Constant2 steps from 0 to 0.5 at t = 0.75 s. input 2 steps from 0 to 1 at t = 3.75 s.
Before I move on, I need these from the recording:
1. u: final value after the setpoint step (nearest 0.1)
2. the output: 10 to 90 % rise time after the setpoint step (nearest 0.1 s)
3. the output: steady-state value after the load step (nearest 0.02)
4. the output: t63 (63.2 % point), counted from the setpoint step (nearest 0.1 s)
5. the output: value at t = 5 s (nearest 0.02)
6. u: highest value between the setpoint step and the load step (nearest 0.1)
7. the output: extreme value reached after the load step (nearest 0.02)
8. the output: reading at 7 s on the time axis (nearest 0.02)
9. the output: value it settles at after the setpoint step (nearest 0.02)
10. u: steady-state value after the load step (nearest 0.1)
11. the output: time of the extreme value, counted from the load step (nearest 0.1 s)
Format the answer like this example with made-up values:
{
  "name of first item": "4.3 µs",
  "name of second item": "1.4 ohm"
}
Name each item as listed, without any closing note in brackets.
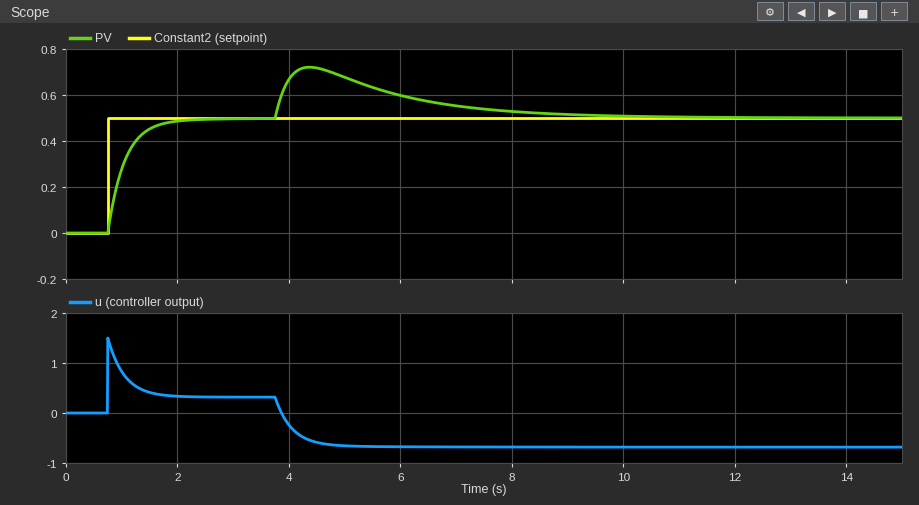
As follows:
{
  "u: final value after the setpoint step": "0.3",
  "the output: 10 to 90 % rise time after the setpoint step": "0.7 s",
  "the output: steady-state value after the load step": "0.50",
  "the output: t63 (63.2 % point), counted from the setpoint step": "0.3 s",
  "the output: value at t = 5 s": "0.68",
  "u: highest value between the setpoint step and the load step": "1.5",
  "the output: extreme value reached after the load step": "0.72",
  "the output: reading at 7 s on the time axis": "0.56",
  "the output: value it settles at after the setpoint step": "0.50",
  "u: steady-state value after the load step": "-0.7",
  "the output: time of the extreme value, counted from the load step": "0.6 s"
}
